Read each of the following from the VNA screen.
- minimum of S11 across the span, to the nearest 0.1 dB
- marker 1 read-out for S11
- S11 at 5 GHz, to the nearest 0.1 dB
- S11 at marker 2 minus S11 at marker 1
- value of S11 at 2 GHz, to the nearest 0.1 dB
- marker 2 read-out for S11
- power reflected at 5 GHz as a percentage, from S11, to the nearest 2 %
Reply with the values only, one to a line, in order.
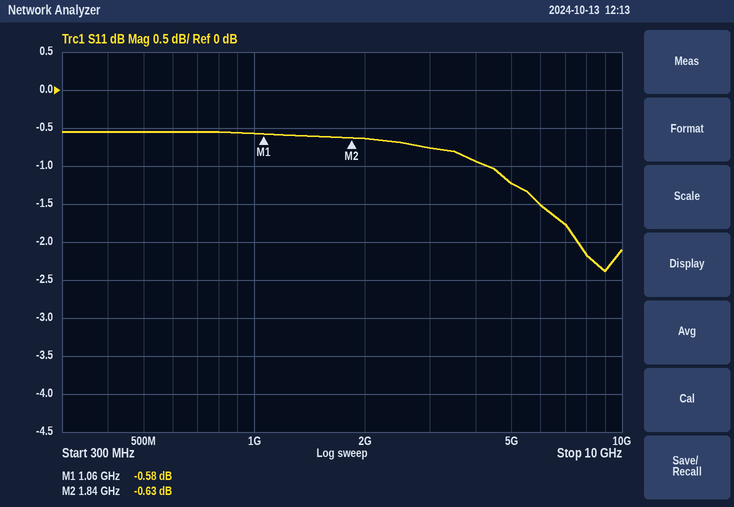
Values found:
-2.4 dB
-0.58 dB
-1.2 dB
-0.05 dB
-0.6 dB
-0.63 dB
76 %
